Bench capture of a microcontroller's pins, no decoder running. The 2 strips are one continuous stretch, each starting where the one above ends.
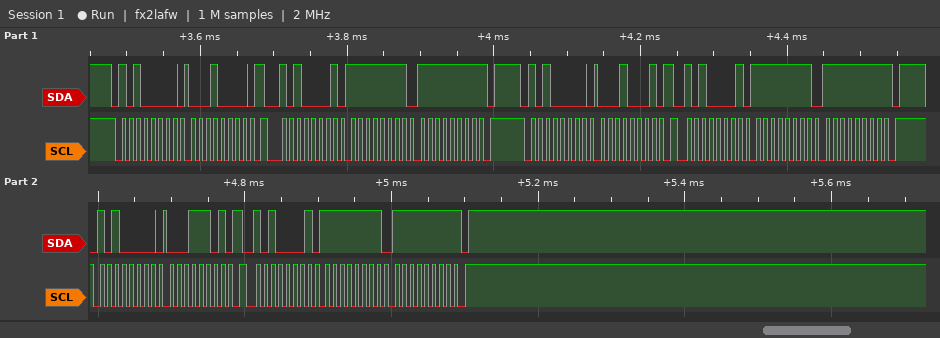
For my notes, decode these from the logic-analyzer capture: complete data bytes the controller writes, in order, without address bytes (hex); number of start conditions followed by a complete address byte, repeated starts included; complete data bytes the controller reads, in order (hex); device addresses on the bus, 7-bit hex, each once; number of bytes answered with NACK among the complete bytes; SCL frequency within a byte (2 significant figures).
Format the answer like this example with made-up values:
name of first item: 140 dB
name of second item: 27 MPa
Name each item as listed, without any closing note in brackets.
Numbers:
complete data bytes the controller writes, in order, without address bytes: 10 11 1D
number of start conditions followed by a complete address byte, repeated starts included: 6
complete data bytes the controller reads, in order: FF FF FF FF FF FF
device addresses on the bus, 7-bit hex, each once: 0x50
number of bytes answered with NACK among the complete bytes: 3
SCL frequency within a byte: 100 kHz
